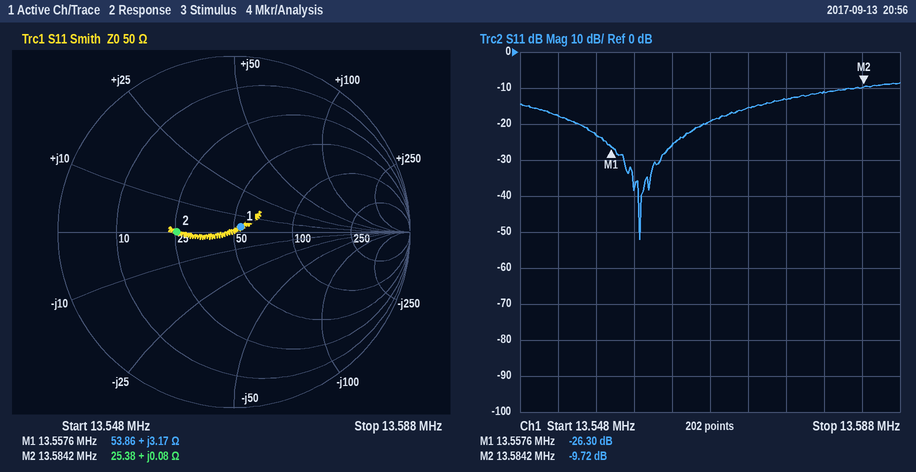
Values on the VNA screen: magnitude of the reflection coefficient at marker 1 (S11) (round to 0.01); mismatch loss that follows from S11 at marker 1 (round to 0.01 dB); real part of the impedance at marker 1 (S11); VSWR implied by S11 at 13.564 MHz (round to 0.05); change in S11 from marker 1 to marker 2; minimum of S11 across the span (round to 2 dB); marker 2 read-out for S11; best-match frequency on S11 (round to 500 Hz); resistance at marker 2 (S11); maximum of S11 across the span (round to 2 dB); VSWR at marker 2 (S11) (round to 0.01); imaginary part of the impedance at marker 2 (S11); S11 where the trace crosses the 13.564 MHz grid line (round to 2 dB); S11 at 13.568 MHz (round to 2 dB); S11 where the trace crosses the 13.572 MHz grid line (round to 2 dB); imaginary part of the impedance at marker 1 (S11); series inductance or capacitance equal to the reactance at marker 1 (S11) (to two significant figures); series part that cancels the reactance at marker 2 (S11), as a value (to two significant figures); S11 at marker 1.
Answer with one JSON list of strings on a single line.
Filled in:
["0.05", "0.01 dB", "53.86 Ω", "1.10", "16.58 dB", "-52 dB", "-9.72 dB", "13.5605 MHz", "25.38 Ω", "-8 dB", "1.97", "+0.08 Ω", "-26 dB", "-20 dB", "-16 dB", "+3.17 Ω", "37 nH", "150 nF", "-26.30 dB"]
